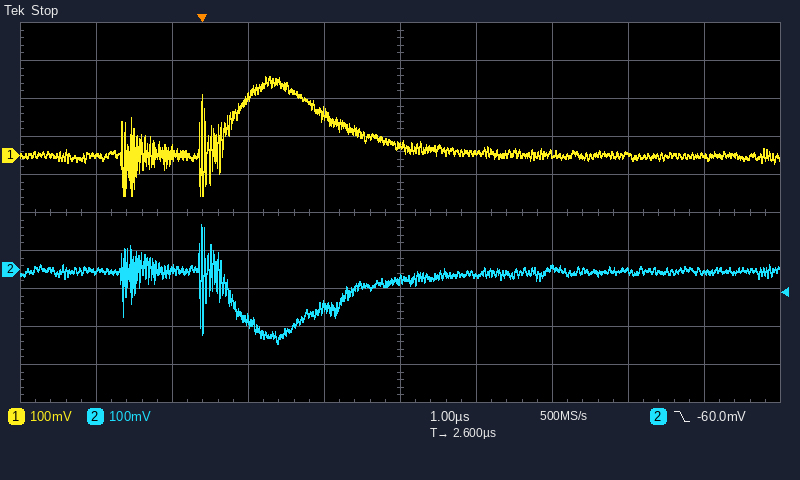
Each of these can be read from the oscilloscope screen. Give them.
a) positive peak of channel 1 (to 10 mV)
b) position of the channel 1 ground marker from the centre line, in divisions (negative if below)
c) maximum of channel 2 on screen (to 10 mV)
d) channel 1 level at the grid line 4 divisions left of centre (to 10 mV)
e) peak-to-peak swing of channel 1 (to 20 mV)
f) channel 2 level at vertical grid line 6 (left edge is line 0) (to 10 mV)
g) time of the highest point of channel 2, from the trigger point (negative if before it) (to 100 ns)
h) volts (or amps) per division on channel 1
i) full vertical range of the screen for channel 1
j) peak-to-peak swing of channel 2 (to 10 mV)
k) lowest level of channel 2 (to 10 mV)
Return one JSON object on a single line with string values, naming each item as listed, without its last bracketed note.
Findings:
{"positive peak of channel 1": "210 mV", "position of the channel 1 ground marker from the centre line, in divisions": "+1.5 div", "maximum of channel 2 on screen": "120 mV", "channel 1 level at the grid line 4 divisions left of centre": "0 mV", "peak-to-peak swing of channel 1": "320 mV", "channel 2 level at vertical grid line 6 (left edge is line 0)": "-10 mV", "time of the highest point of channel 2, from the trigger point (negative if before it)": "0.0 µs", "volts (or amps) per division on channel 1": "100 mV", "full vertical range of the screen for channel 1": "1 V", "peak-to-peak swing of channel 2": "310 mV", "lowest level of channel 2": "-190 mV"}
